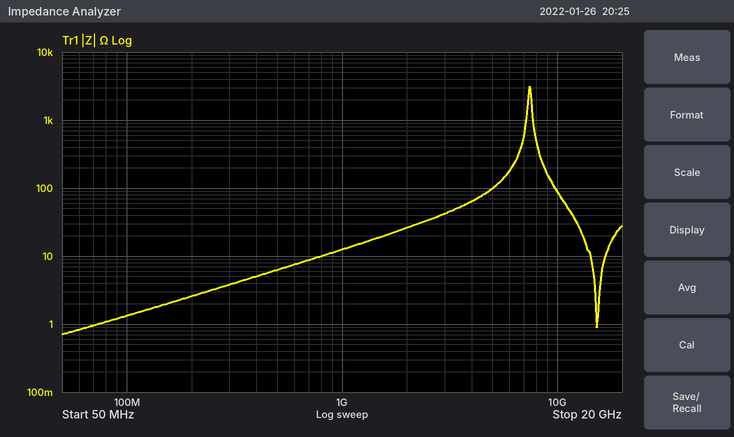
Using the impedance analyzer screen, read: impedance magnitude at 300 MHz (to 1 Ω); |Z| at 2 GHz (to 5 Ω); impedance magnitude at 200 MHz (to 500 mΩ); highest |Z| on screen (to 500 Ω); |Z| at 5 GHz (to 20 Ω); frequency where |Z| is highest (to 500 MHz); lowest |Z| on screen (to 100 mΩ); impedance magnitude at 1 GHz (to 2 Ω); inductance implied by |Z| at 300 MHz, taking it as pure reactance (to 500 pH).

4 Ω
25 Ω
2.5 Ω
3.0 kΩ
100 Ω
7.5 GHz
700 mΩ
12 Ω
2.0 nH
